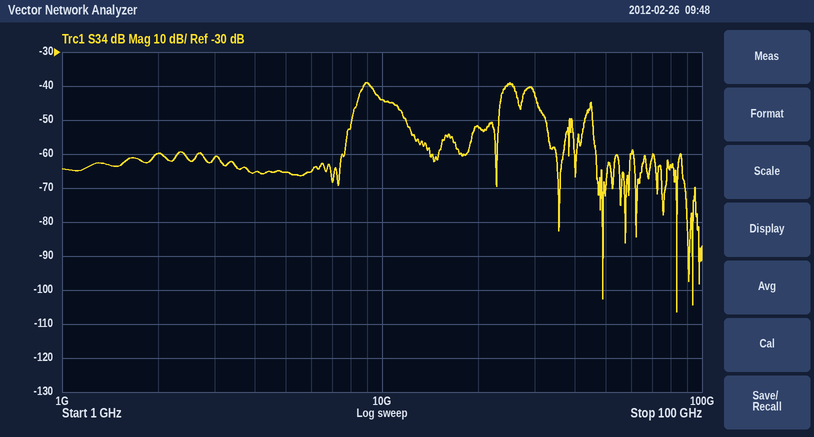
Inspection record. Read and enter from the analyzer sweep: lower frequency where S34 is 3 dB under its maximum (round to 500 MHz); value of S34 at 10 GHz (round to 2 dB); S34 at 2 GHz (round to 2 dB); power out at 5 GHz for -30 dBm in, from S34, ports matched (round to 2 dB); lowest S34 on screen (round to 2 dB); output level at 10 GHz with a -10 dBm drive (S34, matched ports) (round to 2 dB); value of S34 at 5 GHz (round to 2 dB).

8.5 GHz
-44 dB
-60 dB
-96 dBm
-106 dB
-54 dBm
-66 dB
